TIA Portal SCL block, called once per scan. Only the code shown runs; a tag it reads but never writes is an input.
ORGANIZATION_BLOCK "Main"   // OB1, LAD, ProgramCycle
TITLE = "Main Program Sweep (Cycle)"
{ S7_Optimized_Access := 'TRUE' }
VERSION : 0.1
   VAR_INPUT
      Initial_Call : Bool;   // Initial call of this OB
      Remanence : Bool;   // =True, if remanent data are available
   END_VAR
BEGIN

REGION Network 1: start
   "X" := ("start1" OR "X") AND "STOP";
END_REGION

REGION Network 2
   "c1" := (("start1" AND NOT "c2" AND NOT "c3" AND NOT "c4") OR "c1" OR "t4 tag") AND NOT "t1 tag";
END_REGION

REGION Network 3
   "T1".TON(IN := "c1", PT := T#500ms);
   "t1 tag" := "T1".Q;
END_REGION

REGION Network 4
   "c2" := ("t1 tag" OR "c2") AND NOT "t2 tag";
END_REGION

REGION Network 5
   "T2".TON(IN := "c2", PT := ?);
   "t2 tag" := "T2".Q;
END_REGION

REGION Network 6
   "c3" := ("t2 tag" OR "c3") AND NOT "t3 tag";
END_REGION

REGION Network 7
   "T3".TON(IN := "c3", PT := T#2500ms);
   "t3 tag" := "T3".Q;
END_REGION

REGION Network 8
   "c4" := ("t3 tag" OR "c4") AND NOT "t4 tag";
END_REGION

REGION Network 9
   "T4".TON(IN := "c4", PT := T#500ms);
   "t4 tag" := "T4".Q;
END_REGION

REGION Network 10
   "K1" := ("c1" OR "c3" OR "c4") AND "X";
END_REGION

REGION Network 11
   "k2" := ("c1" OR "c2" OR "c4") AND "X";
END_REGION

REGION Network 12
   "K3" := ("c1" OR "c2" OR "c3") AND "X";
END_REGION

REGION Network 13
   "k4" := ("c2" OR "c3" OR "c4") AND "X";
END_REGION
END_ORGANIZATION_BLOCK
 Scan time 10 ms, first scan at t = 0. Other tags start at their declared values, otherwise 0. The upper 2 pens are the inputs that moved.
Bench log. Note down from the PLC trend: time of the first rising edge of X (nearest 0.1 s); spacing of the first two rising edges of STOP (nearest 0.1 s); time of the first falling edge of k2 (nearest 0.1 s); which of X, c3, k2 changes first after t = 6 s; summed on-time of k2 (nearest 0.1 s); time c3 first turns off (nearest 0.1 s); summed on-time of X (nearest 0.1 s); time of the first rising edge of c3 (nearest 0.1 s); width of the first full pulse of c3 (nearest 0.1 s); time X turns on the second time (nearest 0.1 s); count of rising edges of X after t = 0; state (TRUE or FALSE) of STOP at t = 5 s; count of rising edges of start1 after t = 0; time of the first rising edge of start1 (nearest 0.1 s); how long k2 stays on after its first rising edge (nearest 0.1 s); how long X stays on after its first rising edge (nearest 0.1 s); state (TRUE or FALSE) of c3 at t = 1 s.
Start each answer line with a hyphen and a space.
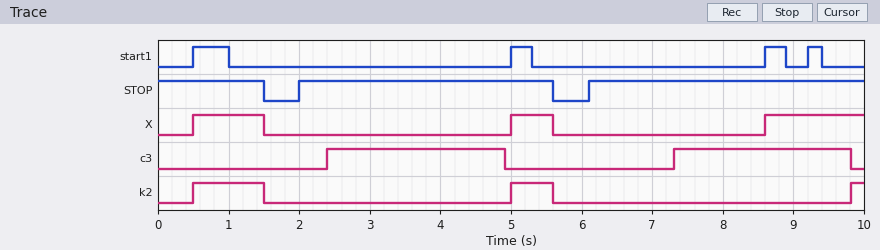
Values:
- 0.5 s
- 4.1 s
- 1.5 s
- c3
- 1.8 s
- 4.9 s
- 3.0 s
- 2.4 s
- 2.5 s
- 5.0 s
- 3
- TRUE
- 4
- 0.5 s
- 1.0 s
- 1.0 s
- FALSE
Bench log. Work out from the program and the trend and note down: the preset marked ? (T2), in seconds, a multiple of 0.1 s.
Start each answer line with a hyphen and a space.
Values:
- 1.4 s
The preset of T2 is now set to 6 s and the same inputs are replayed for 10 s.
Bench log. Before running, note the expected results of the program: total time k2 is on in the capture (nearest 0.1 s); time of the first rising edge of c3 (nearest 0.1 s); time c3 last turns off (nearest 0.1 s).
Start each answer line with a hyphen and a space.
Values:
- 2.1 s
- 7.0 s
- 9.5 s
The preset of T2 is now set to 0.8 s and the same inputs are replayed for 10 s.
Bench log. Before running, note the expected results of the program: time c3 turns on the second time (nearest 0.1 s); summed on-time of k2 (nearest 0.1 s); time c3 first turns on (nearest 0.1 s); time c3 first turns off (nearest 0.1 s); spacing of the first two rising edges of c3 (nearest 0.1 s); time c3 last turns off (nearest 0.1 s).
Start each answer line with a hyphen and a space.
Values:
- 6.1 s
- 3.0 s
- 1.8 s
- 4.3 s
- 4.3 s
- 8.6 s
